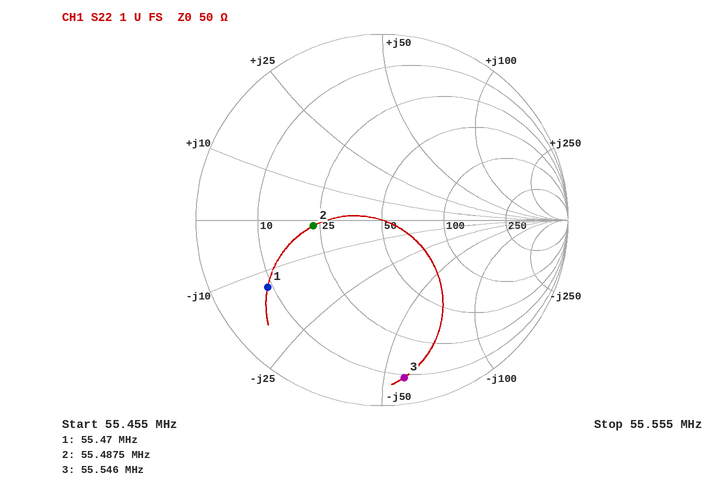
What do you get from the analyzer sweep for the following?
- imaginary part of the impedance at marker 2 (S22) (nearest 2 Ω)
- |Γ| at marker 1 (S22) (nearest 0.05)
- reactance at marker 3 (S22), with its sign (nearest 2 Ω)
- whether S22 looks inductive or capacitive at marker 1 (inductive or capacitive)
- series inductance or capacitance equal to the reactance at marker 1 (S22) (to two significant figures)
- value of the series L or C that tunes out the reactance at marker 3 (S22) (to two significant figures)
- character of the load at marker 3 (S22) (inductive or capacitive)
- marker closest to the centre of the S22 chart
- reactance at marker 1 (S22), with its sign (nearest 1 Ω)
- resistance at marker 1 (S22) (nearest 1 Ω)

-2 Ω
0.70
-56 Ω
capacitive
220 pF
160 nH
capacitive
marker 2
-13 Ω
9 Ω
